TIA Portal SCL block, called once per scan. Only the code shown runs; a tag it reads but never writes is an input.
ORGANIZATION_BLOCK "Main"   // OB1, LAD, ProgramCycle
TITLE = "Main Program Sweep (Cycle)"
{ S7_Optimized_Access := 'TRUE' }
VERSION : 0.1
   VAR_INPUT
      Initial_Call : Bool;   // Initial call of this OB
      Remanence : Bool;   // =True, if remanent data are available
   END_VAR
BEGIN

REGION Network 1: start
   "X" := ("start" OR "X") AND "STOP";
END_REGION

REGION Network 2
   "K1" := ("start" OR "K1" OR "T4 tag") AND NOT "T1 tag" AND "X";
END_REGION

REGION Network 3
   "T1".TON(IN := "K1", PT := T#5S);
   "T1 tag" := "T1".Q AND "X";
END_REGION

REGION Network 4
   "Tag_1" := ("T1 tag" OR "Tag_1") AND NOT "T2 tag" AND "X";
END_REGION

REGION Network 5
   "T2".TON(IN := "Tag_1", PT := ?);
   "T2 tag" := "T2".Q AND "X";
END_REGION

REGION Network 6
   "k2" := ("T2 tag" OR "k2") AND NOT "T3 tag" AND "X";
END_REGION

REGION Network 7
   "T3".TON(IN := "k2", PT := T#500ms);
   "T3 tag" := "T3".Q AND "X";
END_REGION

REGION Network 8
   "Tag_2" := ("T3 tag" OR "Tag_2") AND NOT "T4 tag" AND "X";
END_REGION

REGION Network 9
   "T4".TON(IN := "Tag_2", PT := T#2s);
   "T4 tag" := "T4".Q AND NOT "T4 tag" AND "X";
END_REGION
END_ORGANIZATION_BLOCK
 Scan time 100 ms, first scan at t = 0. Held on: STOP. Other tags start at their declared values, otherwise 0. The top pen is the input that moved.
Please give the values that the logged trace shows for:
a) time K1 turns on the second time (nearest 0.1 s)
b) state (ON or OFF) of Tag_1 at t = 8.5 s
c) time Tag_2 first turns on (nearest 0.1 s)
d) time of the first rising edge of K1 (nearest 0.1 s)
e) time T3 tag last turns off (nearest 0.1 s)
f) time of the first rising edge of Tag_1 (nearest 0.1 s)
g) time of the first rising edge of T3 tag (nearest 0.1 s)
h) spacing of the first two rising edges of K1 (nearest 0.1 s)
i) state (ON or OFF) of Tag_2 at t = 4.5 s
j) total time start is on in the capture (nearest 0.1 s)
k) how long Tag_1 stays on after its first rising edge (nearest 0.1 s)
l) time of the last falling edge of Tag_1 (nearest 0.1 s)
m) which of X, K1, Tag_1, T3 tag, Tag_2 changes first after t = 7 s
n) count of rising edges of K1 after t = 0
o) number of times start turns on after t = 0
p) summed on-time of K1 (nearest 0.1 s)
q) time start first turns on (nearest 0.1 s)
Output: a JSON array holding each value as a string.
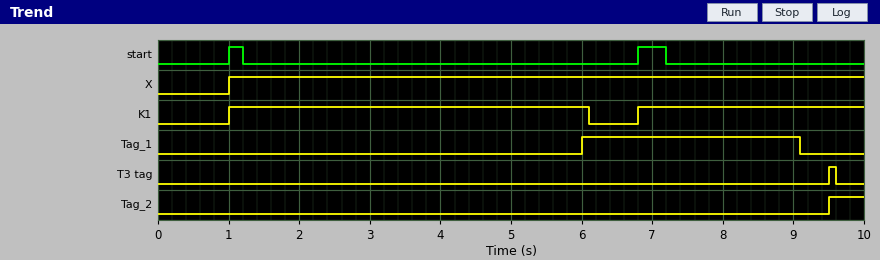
["6.8 s", "ON", "9.5 s", "1.0 s", "9.6 s", "6.0 s", "9.5 s", "5.8 s", "OFF", "0.6 s", "3.1 s", "9.1 s", "Tag_1", "2", "2", "8.3 s", "1.0 s"]
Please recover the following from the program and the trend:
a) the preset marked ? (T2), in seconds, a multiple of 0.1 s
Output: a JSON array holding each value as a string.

["3.0 s"]
